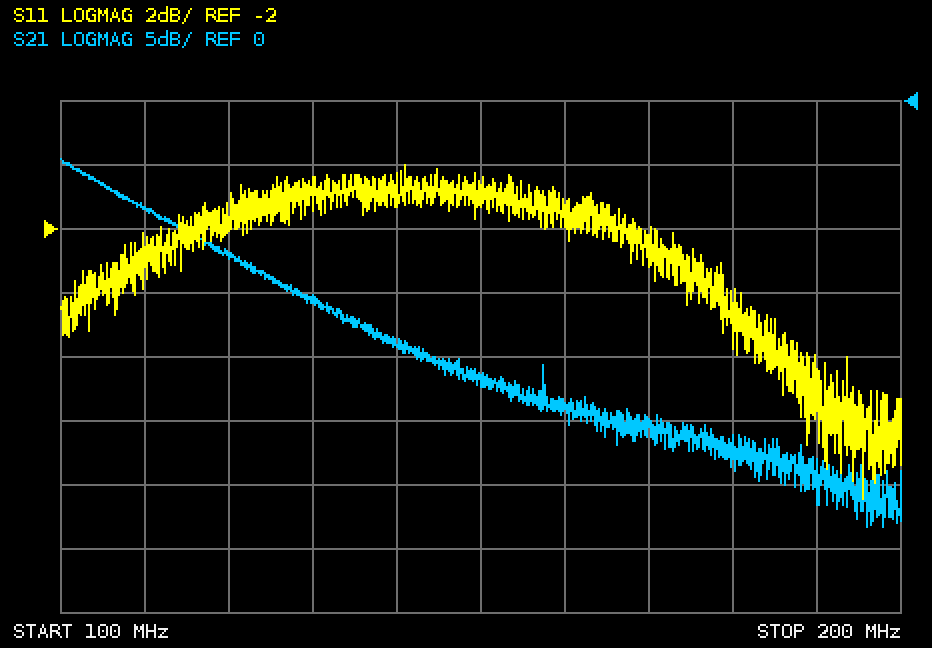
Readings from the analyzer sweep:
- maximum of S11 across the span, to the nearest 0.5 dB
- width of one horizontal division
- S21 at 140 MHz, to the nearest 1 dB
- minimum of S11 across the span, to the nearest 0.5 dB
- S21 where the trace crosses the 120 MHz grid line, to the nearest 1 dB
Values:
0.0 dB
10 MHz
-19 dB
-10.5 dB
-12 dB
